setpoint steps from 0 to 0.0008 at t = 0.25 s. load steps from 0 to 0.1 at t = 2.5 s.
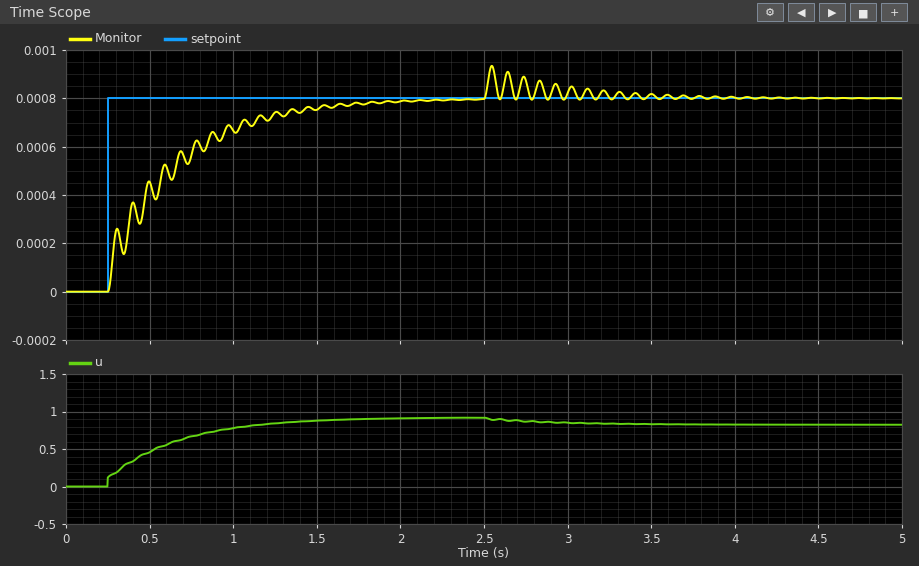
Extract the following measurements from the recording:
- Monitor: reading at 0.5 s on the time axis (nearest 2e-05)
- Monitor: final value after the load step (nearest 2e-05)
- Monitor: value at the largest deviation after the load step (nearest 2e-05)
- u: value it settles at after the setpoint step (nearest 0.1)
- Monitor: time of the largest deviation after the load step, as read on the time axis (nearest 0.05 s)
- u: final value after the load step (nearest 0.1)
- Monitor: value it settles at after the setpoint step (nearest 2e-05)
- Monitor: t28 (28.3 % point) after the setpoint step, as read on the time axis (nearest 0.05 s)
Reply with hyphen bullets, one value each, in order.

- 0.00046
- 0.00080
- 0.00094
- 0.9
- 2.55 s
- 0.8
- 0.00080
- 0.30 s
